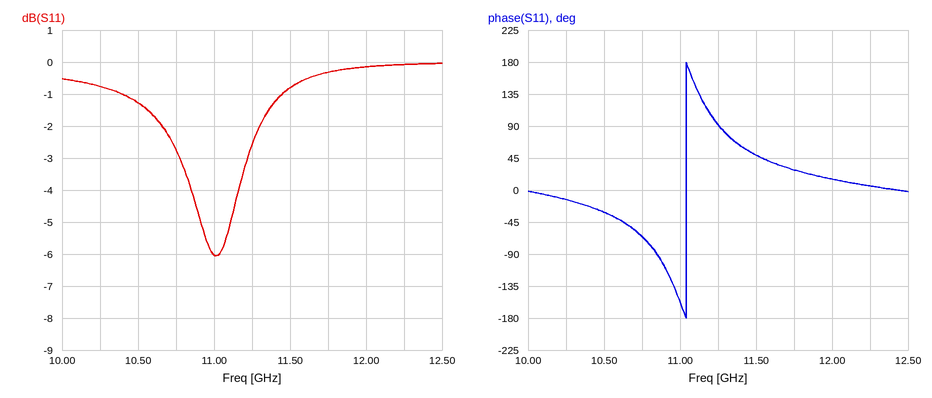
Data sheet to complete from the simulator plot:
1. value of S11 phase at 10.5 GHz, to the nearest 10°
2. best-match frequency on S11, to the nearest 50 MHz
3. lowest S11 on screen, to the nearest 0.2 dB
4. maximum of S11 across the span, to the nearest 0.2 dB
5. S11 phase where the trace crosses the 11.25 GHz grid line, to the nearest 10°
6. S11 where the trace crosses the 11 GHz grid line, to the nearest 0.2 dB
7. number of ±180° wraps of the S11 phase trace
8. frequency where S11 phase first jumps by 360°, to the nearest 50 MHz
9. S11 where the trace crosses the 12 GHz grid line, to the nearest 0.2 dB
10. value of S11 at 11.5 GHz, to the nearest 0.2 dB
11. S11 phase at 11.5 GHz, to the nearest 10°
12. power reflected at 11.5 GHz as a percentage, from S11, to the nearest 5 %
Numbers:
-30°
11.00 GHz
-6.0 dB
0.0 dB
90°
-6.0 dB
1
11.05 GHz
-0.2 dB
-0.8 dB
50°
85 %
